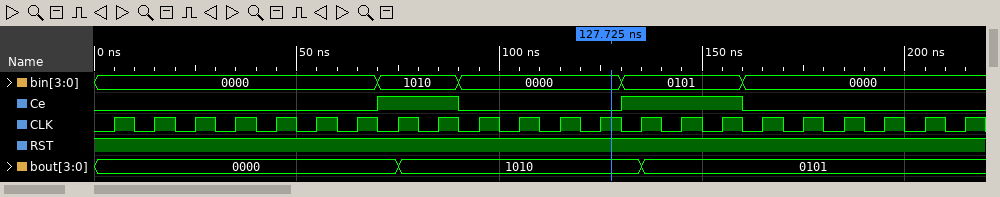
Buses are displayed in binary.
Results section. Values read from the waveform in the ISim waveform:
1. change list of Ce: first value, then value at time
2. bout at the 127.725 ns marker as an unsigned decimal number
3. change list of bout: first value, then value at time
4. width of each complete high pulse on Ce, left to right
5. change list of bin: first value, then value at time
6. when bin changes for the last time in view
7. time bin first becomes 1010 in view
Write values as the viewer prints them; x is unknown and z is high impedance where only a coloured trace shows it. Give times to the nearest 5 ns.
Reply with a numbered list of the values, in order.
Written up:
1. 0, 1 at 70 ns, 0 at 90 ns, 1 at 130 ns, 0 at 160 ns
2. 10
3. 0000, 1010 at 75 ns, 0101 at 135 ns
4. 20 ns, 30 ns
5. 0000, 1010 at 70 ns, 0000 at 90 ns, 0101 at 130 ns, 0000 at 160 ns
6. 160 ns
7. 70 ns
